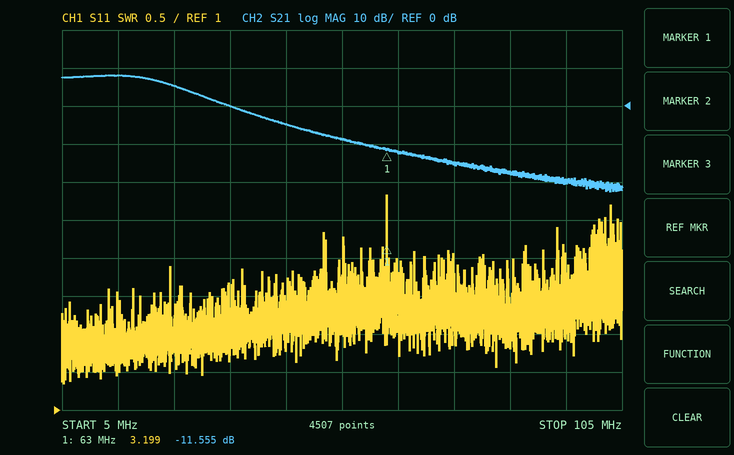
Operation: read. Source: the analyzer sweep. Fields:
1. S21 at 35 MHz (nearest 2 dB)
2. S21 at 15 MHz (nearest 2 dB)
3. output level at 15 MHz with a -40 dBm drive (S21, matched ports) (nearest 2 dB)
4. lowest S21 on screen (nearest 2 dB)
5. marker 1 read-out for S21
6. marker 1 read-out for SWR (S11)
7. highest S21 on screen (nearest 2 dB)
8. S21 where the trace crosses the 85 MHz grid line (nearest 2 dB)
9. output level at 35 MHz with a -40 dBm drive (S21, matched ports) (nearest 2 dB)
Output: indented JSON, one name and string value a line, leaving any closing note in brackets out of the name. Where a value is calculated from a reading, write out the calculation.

{
  "S21 at 35 MHz": "0 dB",
  "S21 at 15 MHz": "8 dB",
  "output level at 15 MHz with a -40 dBm drive (S21, matched ports)": "-40 dBm + (8 dB) = -32 dBm",
  "lowest S21 on screen": "-22 dB",
  "marker 1 read-out for S21": "-11.555 dB",
  "marker 1 read-out for SWR": "3.199",
  "highest S21 on screen": "8 dB",
  "S21 where the trace crosses the 85 MHz grid line": "-18 dB",
  "output level at 35 MHz with a -40 dBm drive (S21, matched ports)": "-40 dBm + (0 dB) = -40 dBm"
}
